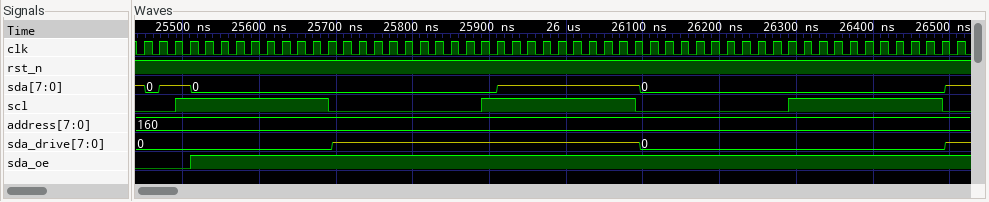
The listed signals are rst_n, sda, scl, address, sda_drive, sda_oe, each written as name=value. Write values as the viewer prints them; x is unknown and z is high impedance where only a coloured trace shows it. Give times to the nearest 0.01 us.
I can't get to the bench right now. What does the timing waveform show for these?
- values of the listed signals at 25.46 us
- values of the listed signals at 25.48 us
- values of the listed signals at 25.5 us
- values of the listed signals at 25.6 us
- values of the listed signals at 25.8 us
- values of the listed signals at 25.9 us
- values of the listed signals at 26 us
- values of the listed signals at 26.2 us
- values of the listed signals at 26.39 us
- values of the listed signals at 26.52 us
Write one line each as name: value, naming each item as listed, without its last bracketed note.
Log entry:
values of the listed signals at 25.46 us: rst_n=1, sda=0, scl=0, address=160, sda_drive=0, sda_oe=0
values of the listed signals at 25.48 us: rst_n=1, sda=z, scl=0, address=160, sda_drive=0, sda_oe=0
values of the listed signals at 25.5 us: rst_n=1, sda=z, scl=1, address=160, sda_drive=0, sda_oe=0
values of the listed signals at 25.6 us: rst_n=1, sda=0, scl=1, address=160, sda_drive=0, sda_oe=1
values of the listed signals at 25.8 us: rst_n=1, sda=0, scl=0, address=160, sda_drive=z, sda_oe=1
values of the listed signals at 25.9 us: rst_n=1, sda=0, scl=1, address=160, sda_drive=z, sda_oe=1
values of the listed signals at 26 us: rst_n=1, sda=z, scl=1, address=160, sda_drive=z, sda_oe=1
values of the listed signals at 26.2 us: rst_n=1, sda=0, scl=0, address=160, sda_drive=0, sda_oe=1
values of the listed signals at 26.39 us: rst_n=1, sda=0, scl=1, address=160, sda_drive=0, sda_oe=1
values of the listed signals at 26.52 us: rst_n=1, sda=z, scl=0, address=160, sda_drive=z, sda_oe=1
